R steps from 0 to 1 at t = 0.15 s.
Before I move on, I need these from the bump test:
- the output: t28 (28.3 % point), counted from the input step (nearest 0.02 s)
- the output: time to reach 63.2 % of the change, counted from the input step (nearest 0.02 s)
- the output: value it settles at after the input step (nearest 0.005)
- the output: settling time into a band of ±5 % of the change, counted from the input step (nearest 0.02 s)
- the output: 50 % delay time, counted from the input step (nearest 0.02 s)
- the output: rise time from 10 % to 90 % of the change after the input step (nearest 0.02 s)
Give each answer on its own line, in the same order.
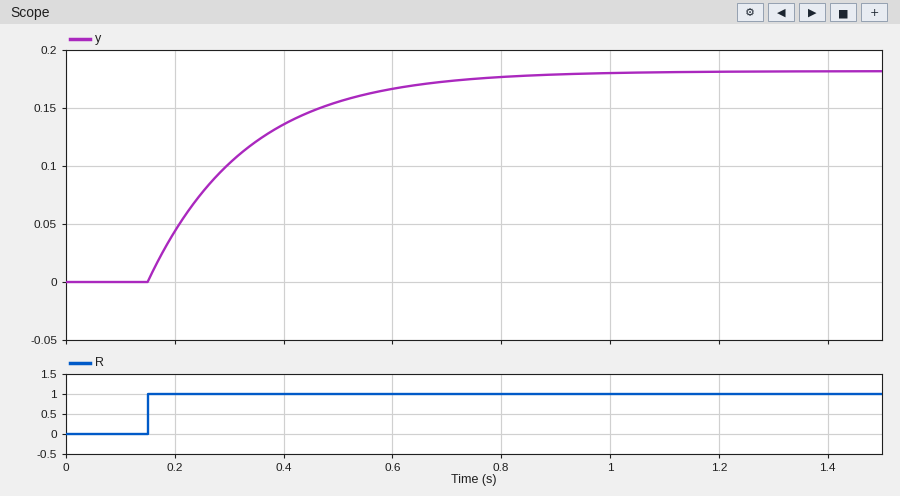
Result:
0.06 s
0.18 s
0.180
0.54 s
0.12 s
0.40 s
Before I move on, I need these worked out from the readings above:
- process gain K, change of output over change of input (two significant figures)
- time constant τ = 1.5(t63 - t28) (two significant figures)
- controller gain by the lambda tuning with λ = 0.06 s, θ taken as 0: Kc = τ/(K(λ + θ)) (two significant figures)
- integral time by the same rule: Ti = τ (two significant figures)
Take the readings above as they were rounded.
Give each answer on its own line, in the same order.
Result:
0.18
0.18 s
17
0.18 s
